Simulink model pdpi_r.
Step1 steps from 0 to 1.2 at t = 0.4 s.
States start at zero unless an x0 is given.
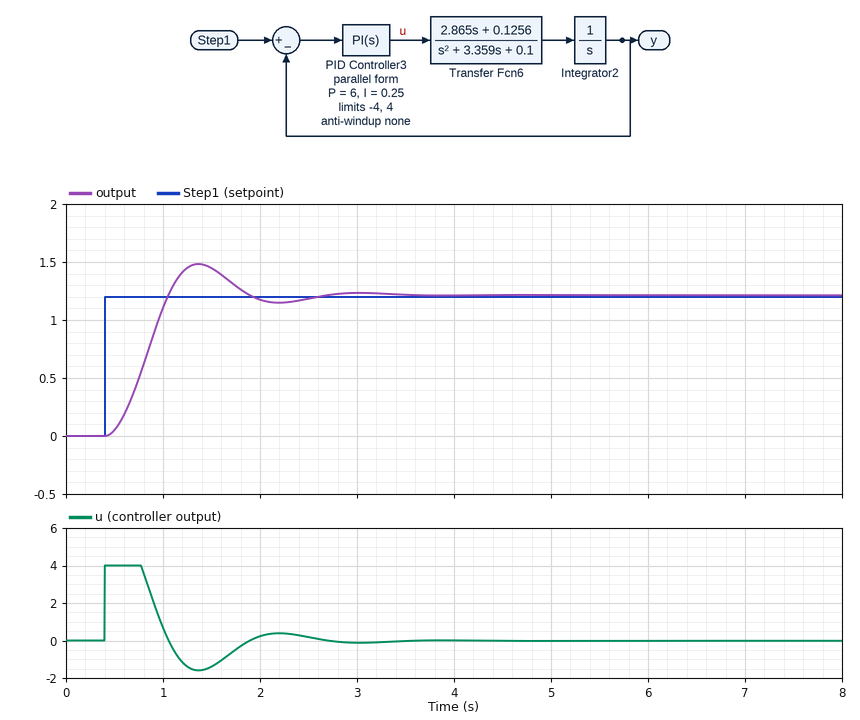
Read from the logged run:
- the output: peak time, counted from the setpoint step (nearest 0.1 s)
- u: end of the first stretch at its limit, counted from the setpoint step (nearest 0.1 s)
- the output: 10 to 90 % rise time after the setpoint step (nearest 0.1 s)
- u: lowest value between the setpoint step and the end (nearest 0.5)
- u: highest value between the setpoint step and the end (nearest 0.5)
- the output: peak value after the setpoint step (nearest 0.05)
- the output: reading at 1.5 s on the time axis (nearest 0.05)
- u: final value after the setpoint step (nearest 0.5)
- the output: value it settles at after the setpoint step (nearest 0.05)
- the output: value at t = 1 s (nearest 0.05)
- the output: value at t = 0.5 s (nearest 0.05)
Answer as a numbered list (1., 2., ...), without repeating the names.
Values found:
1. 1.0 s
2. 0.4 s
3. 0.4 s
4. -1.5
5. 4.0
6. 1.50
7. 1.45
8. 0.0
9. 1.20
10. 1.10
11. 0.05
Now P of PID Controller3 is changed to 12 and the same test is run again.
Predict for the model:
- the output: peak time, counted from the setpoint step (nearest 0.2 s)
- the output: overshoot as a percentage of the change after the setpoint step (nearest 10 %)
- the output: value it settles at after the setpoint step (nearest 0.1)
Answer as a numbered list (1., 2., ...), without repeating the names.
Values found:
1. 0.8 s
2. 20 %
3. 1.2
